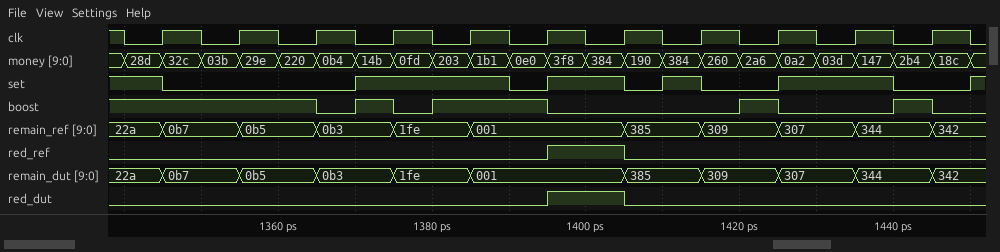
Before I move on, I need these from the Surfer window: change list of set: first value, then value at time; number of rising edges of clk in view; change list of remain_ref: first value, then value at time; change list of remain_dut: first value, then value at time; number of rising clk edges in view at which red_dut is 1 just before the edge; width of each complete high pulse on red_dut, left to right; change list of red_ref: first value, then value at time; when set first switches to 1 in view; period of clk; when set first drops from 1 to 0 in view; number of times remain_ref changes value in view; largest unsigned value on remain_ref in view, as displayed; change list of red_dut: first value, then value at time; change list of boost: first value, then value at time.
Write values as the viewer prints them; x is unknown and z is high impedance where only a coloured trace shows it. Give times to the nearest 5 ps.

1, 0 at 1345 ps, 1 at 1370 ps, 0 at 1390 ps, 1 at 1395 ps, 0 at 1405 ps, 1 at 1410 ps, 0 at 1415 ps, 1 at 1425 ps, 0 at 1440 ps, 1 at 1450 ps
11
22a, 0b7 at 1345 ps, 0b5 at 1355 ps, 0b3 at 1365 ps, 1fe at 1375 ps, 001 at 1385 ps, 385 at 1405 ps, 309 at 1415 ps, 307 at 1425 ps, 344 at 1435 ps, 342 at 1445 ps
22a, 0b7 at 1345 ps, 0b5 at 1355 ps, 0b3 at 1365 ps, 1fe at 1375 ps, 001 at 1385 ps, 385 at 1405 ps, 309 at 1415 ps, 307 at 1425 ps, 344 at 1435 ps, 342 at 1445 ps
1
10 ps
0, 1 at 1395 ps, 0 at 1405 ps
1370 ps
10 ps
1345 ps
10
385
0, 1 at 1395 ps, 0 at 1405 ps
1, 0 at 1365 ps, 1 at 1370 ps, 0 at 1375 ps, 1 at 1380 ps, 0 at 1395 ps, 1 at 1420 ps, 0 at 1425 ps, 1 at 1440 ps, 0 at 1445 ps
